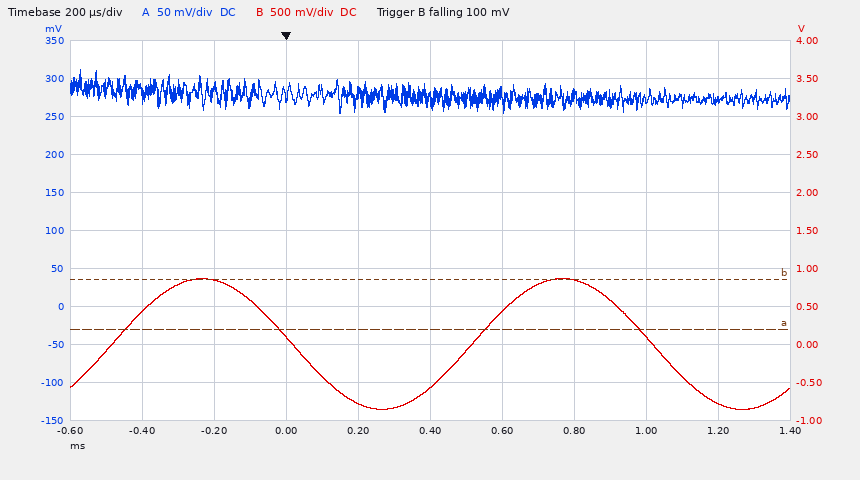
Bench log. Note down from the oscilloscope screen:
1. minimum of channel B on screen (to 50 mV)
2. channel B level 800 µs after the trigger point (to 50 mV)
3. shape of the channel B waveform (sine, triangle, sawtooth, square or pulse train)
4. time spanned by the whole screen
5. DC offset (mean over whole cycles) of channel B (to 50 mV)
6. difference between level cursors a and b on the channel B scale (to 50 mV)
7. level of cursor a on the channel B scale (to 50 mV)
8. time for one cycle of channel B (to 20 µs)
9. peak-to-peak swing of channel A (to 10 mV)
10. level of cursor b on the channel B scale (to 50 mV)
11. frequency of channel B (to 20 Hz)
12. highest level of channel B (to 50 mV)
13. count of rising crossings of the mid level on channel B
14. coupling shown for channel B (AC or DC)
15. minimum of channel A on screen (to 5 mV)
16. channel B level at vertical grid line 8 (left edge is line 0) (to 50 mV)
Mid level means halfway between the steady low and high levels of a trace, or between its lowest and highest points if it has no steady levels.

-850 mV
850 mV
sine
2 ms
0 mV
650 mV
200 mV
1.00 ms
60 mV
850 mV
1.00 kHz
850 mV
2
DC
255 mV
100 mV
